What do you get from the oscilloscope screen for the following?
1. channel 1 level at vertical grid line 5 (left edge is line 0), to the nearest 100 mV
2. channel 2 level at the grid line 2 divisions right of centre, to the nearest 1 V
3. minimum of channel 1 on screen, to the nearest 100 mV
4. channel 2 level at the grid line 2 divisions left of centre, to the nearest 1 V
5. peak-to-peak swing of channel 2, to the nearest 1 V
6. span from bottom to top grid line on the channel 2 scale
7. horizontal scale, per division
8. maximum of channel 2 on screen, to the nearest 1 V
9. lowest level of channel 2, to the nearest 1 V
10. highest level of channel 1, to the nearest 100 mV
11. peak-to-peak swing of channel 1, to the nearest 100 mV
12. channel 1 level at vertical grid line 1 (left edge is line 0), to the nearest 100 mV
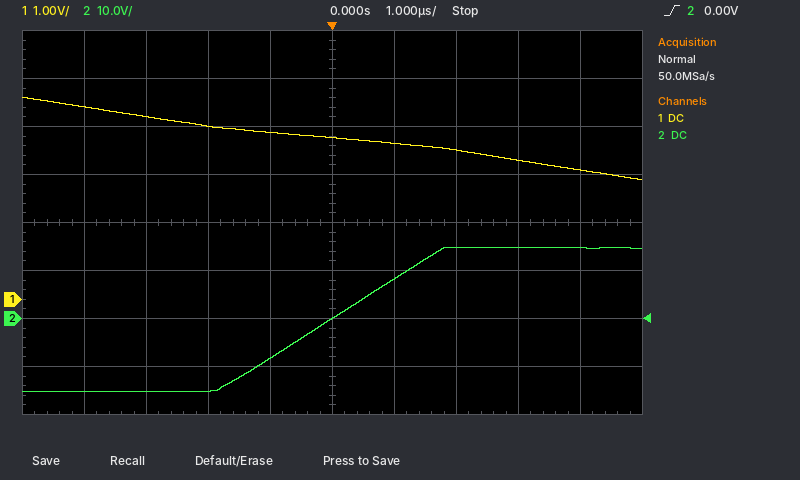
3.4 V
15 V
2.5 V
-15 V
30 V
80 V
1 µs
15 V
-15 V
4.2 V
1.7 V
4.0 V
